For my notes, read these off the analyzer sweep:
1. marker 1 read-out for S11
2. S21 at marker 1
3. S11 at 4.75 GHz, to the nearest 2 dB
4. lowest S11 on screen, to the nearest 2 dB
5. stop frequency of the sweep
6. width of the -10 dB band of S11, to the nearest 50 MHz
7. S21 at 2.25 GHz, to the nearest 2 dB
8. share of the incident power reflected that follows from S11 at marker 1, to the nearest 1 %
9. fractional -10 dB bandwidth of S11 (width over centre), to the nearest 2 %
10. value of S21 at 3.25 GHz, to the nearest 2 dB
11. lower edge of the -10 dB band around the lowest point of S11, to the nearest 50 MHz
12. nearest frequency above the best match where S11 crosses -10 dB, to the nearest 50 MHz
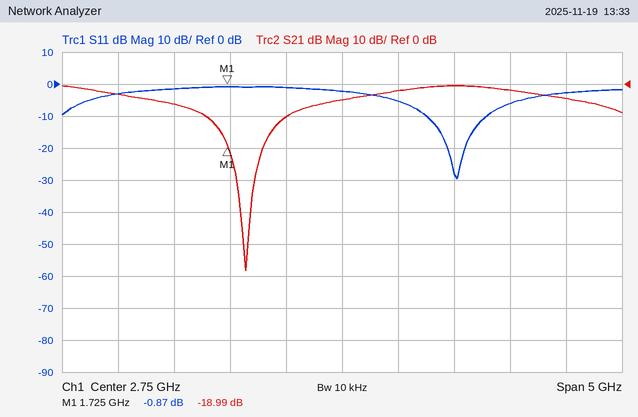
-0.87 dB
-18.99 dB
-2 dB
-30 dB
5.25 GHz
550 MHz
-10 dB
82 %
14 %
-2 dB
3.50 GHz
4.05 GHz
